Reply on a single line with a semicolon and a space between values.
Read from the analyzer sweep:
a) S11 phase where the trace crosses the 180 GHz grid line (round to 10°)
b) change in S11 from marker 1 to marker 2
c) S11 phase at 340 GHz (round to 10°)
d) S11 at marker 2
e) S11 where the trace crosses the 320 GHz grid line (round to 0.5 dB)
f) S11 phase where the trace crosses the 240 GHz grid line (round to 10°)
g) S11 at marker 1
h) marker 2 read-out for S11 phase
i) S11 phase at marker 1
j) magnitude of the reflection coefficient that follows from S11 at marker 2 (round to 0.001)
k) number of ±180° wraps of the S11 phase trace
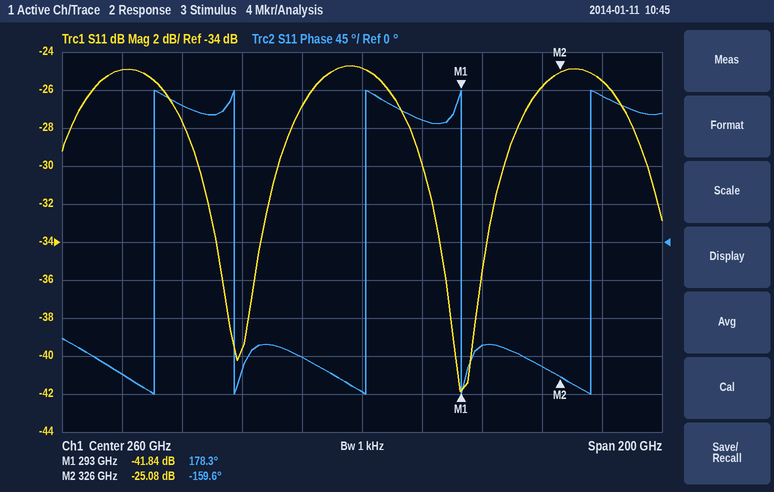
-160°; 16.76 dB; 170°; -25.08 dB; -26.0 dB; -140°; -41.84 dB; -159.6°; 178.3°; 0.056; 5
